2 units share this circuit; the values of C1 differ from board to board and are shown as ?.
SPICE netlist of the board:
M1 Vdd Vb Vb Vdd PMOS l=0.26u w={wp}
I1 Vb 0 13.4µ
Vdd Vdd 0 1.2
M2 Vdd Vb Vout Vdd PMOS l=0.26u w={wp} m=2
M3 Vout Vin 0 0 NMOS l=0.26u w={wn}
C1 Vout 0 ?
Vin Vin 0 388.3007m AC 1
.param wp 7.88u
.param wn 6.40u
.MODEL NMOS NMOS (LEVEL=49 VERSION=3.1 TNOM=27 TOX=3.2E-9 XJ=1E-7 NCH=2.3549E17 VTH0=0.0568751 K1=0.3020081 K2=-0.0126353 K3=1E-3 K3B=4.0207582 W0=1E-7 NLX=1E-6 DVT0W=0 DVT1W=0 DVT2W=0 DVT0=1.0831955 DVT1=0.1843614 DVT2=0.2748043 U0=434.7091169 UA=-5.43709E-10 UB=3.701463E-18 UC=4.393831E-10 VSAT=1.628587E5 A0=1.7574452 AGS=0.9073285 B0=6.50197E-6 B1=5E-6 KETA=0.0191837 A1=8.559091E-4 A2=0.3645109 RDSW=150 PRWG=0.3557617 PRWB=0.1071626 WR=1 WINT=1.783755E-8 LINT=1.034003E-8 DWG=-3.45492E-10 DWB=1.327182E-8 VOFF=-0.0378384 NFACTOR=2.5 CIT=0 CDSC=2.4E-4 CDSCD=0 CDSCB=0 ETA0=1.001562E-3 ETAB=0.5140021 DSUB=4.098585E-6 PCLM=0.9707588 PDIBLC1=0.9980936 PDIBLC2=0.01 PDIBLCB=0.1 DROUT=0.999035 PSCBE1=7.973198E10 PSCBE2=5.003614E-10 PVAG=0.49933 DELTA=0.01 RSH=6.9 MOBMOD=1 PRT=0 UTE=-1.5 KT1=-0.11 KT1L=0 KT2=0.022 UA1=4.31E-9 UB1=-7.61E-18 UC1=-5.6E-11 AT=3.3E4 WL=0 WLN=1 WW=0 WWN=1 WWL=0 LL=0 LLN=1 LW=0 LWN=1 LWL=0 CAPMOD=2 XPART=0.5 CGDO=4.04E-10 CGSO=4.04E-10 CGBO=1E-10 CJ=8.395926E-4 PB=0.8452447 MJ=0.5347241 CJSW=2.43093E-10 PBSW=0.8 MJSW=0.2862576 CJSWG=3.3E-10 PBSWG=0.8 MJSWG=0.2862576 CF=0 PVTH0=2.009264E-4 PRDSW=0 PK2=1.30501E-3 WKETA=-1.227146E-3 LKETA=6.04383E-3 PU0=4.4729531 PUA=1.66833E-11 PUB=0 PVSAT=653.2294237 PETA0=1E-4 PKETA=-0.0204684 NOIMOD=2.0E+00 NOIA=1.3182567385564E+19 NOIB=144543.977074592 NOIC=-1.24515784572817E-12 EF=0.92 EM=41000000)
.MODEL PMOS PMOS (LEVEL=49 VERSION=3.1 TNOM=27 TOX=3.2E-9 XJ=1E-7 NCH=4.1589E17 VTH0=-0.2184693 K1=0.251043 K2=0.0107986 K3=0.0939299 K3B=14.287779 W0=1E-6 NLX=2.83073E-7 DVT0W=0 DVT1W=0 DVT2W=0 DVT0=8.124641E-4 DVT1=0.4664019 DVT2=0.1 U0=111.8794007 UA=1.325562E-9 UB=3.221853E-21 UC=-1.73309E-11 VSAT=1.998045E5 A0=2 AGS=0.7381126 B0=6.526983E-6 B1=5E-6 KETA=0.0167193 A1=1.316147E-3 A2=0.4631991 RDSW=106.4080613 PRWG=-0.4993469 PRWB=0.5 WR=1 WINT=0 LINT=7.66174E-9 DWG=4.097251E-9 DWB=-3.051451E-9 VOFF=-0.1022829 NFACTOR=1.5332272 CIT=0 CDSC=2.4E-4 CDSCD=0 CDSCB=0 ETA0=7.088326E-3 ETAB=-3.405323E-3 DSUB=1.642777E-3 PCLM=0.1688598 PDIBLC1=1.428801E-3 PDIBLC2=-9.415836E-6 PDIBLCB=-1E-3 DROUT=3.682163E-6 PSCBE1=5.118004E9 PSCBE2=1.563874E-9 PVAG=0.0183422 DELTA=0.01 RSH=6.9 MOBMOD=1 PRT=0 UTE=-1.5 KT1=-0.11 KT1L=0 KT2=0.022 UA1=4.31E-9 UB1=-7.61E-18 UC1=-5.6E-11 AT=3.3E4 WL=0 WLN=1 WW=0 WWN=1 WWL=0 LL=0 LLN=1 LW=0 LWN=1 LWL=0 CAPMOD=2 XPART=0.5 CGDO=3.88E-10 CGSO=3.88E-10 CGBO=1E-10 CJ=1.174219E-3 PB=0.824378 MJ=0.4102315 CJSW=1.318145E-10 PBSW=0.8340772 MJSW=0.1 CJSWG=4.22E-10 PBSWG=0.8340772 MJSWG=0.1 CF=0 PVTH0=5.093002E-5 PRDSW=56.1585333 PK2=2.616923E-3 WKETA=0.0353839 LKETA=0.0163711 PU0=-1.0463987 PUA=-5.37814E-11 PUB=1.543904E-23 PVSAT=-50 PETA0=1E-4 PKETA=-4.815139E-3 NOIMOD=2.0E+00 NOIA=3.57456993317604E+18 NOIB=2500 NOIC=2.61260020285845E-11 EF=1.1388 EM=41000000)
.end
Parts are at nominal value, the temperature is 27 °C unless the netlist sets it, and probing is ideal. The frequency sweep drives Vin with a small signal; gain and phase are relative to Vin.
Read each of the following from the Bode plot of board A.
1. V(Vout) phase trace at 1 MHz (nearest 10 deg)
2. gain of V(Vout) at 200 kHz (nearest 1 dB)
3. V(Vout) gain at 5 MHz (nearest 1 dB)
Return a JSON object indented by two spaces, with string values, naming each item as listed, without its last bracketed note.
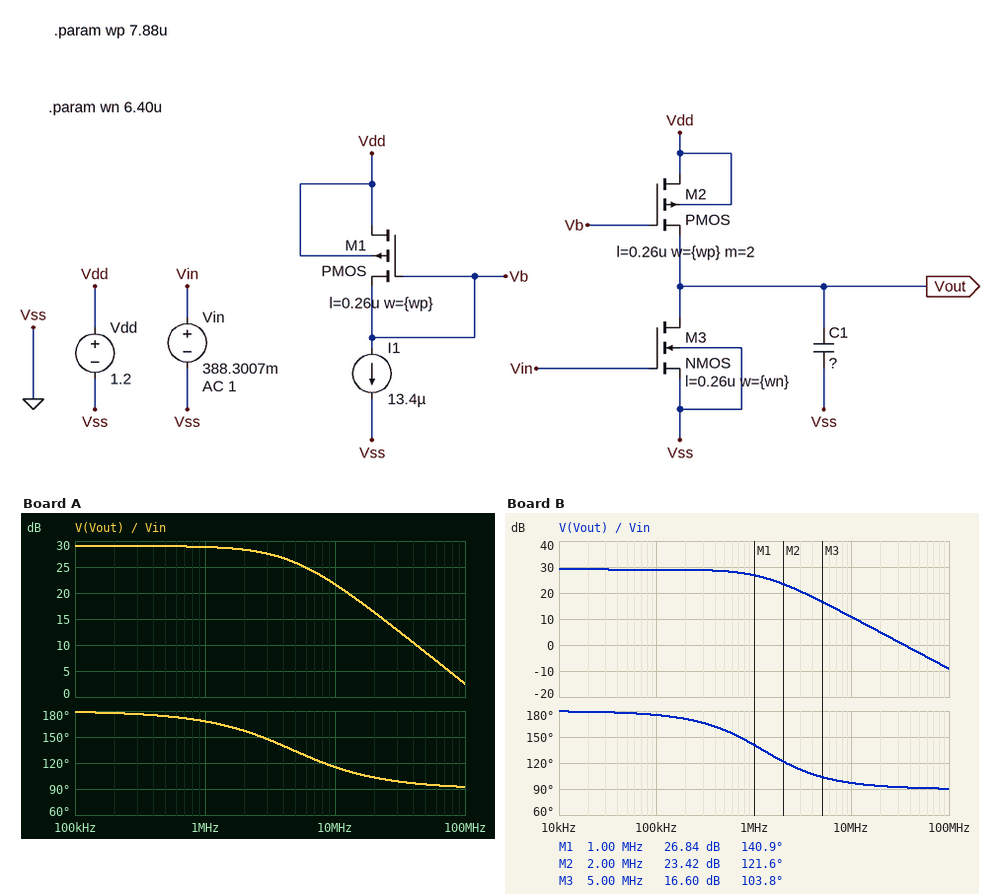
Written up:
{
  "V(Vout) phase trace at 1 MHz": "170 deg",
  "gain of V(Vout) at 200 kHz": "29 dB",
  "V(Vout) gain at 5 MHz": "26 dB"
}
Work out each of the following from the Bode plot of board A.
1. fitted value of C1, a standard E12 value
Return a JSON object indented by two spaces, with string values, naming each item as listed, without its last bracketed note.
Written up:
{
  "fitted value of C1, a standard E12 value": "680 fF"
}
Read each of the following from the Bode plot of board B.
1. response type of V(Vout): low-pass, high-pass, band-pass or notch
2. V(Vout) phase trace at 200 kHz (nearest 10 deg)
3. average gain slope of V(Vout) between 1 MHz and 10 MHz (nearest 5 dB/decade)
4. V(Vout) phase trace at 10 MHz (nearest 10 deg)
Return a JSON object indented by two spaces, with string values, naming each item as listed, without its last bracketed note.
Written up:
{
  "response type of V(Vout): low-pass, high-pass, band-pass or notch": "low-pass",
  "V(Vout) phase trace at 200 kHz": "170 deg",
  "average gain slope of V(Vout) between 1 MHz and 10 MHz": "-15 dB/decade",
  "V(Vout) phase trace at 10 MHz": "100 deg"
}
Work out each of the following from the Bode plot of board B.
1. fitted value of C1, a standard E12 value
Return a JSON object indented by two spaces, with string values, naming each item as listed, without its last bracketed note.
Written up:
{
  "fitted value of C1, a standard E12 value": "2.7 pF"
}
